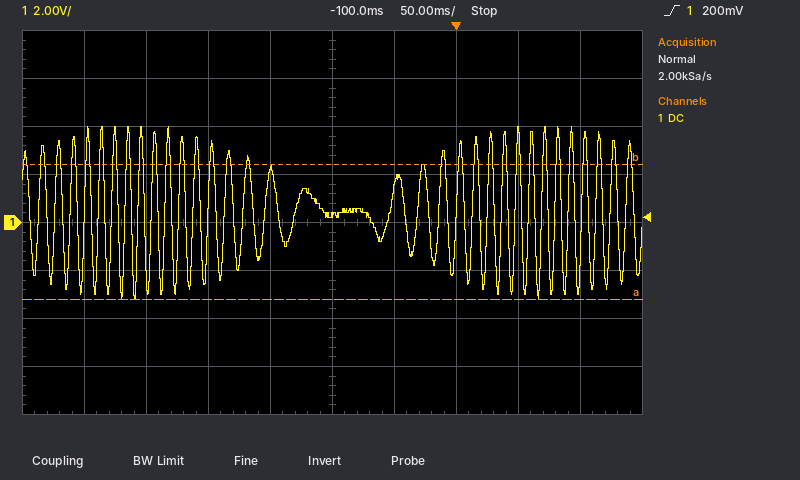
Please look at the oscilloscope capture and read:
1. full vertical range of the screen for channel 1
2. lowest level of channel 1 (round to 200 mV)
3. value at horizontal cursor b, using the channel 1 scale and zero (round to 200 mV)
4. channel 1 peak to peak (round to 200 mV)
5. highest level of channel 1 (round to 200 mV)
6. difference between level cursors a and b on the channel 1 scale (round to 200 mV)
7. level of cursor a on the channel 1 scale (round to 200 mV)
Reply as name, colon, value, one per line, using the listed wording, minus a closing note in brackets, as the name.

full vertical range of the screen for channel 1: 16 V
lowest level of channel 1: -3.2 V
value at horizontal cursor b, using the channel 1 scale and zero: 2.4 V
channel 1 peak to peak: 7.2 V
highest level of channel 1: 4.0 V
difference between level cursors a and b on the channel 1 scale: 5.6 V
level of cursor a on the channel 1 scale: -3.2 V
